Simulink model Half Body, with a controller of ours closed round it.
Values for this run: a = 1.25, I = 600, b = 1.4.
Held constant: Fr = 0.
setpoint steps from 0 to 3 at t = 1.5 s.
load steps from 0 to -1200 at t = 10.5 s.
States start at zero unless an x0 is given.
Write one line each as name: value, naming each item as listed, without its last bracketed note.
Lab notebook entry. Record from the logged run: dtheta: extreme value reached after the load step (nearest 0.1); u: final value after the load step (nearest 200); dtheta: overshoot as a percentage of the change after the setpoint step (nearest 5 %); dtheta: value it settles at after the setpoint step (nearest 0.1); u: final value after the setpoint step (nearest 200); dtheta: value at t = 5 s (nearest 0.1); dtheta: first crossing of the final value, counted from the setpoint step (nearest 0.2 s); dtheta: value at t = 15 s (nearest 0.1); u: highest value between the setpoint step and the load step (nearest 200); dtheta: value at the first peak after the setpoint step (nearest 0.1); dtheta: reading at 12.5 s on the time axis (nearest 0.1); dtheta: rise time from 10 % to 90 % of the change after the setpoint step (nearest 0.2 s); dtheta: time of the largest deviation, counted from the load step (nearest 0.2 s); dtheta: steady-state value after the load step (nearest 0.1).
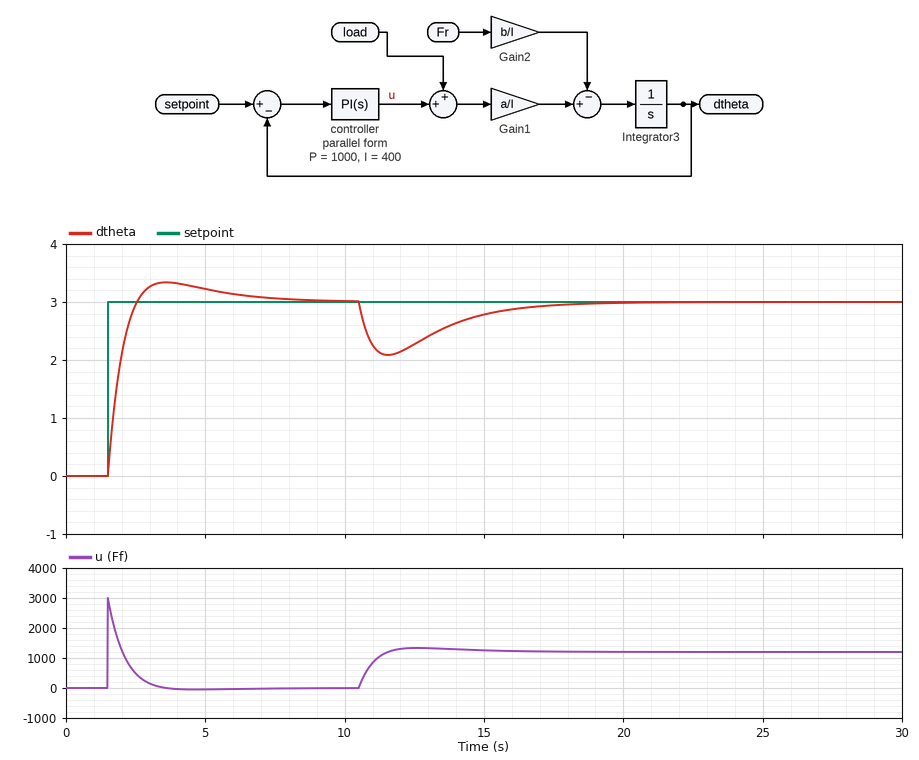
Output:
dtheta: extreme value reached after the load step: 2.1
u: final value after the load step: 1200
dtheta: overshoot as a percentage of the change after the setpoint step: 10 %
dtheta: value it settles at after the setpoint step: 3.0
u: final value after the setpoint step: 0
dtheta: value at t = 5 s: 3.2
dtheta: first crossing of the final value, counted from the setpoint step: 1.0 s
dtheta: value at t = 15 s: 2.8
u: highest value between the setpoint step and the load step: 3000
dtheta: value at the first peak after the setpoint step: 3.3
dtheta: reading at 12.5 s on the time axis: 2.3
dtheta: rise time from 10 % to 90 % of the change after the setpoint step: 0.8 s
dtheta: time of the largest deviation, counted from the load step: 1.0 s
dtheta: steady-state value after the load step: 3.0
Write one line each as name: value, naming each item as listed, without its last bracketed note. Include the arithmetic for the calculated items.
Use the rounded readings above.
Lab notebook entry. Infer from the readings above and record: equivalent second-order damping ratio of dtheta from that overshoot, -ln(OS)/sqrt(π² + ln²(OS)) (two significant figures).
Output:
equivalent second-order damping ratio of dtheta from that overshoot, -ln(OS)/sqrt(π² + ln²(OS)): ln(0.1) = -2.303; 2.303 / sqrt(9.870 + 5.302) = 0.59
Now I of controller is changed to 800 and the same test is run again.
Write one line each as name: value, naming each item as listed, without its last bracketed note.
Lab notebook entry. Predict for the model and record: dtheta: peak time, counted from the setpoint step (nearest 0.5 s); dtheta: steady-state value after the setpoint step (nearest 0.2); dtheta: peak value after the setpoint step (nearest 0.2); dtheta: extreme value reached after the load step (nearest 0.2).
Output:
dtheta: peak time, counted from the setpoint step: 1.5 s
dtheta: steady-state value after the setpoint step: 3.0
dtheta: peak value after the setpoint step: 3.6
dtheta: extreme value reached after the load step: 2.2
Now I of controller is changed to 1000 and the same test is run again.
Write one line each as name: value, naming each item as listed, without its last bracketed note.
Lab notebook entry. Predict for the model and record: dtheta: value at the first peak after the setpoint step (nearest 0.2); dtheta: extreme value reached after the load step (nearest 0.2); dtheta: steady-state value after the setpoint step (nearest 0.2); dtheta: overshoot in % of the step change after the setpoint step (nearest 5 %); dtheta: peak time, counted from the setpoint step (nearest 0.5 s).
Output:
dtheta: value at the first peak after the setpoint step: 3.6
dtheta: extreme value reached after the load step: 2.2
dtheta: steady-state value after the setpoint step: 3.0
dtheta: overshoot in % of the step change after the setpoint step: 20 %
dtheta: peak time, counted from the setpoint step: 1.5 s
